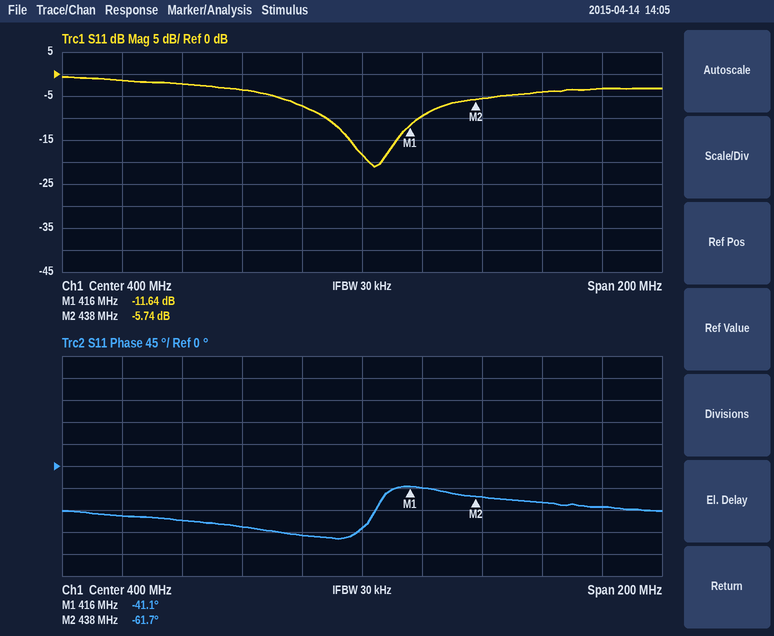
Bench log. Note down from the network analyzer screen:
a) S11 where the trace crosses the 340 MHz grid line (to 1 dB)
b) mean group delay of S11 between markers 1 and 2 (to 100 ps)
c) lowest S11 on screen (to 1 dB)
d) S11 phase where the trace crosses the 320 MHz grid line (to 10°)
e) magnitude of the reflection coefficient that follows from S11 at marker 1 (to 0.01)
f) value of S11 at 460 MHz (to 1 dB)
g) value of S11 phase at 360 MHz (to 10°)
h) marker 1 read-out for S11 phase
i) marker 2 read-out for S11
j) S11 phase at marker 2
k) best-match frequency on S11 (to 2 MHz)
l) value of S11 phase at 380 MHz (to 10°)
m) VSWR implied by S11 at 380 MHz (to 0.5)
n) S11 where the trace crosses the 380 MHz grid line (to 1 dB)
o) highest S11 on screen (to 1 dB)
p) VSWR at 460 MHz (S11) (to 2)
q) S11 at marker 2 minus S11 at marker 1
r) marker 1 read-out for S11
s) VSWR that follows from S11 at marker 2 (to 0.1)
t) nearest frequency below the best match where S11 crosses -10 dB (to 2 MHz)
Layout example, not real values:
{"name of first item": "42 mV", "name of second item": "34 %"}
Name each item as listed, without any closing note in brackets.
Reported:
{"S11 where the trace crosses the 340 MHz grid line": "-2 dB", "mean group delay of S11 between markers 1 and 2": "2.6 ns", "lowest S11 on screen": "-21 dB", "S11 phase where the trace crosses the 320 MHz grid line": "-100°", "magnitude of the reflection coefficient that follows from S11 at marker 1": "0.26", "value of S11 at 460 MHz": "-4 dB", "value of S11 phase at 360 MHz": "-120°", "marker 1 read-out for S11 phase": "-41.1°", "marker 2 read-out for S11": "-5.74 dB", "S11 phase at marker 2": "-61.7°", "best-match frequency on S11": "404 MHz", "value of S11 phase at 380 MHz": "-140°", "VSWR implied by S11 at 380 MHz": "2.5", "S11 where the trace crosses the 380 MHz grid line": "-7 dB", "highest S11 on screen": "-1 dB", "VSWR at 460 MHz (S11)": "4", "S11 at marker 2 minus S11 at marker 1": "5.90 dB", "marker 1 read-out for S11": "-11.64 dB", "VSWR that follows from S11 at marker 2": "3.1", "nearest frequency below the best match where S11 crosses -10 dB": "388 MHz"}
